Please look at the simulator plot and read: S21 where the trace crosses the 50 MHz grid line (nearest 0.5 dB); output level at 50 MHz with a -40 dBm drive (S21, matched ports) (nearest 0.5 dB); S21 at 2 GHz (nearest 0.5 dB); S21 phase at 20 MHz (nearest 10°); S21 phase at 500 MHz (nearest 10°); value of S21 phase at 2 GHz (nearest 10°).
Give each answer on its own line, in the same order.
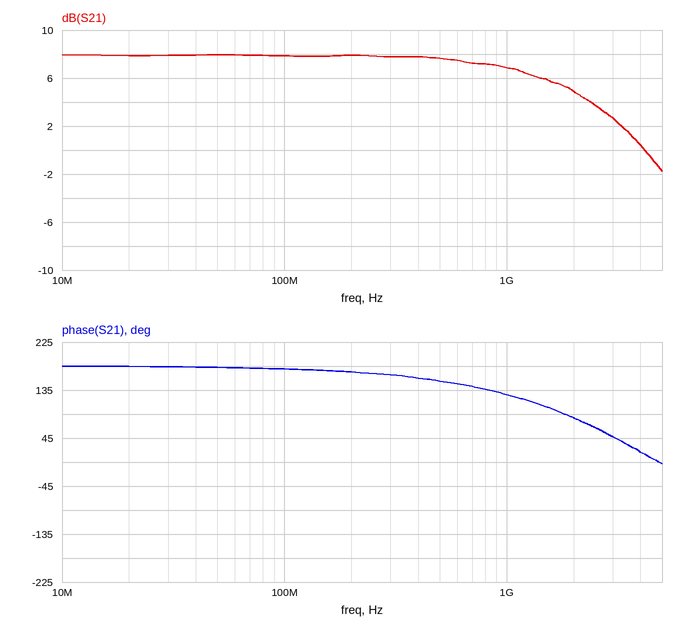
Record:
8.0 dB
-32.0 dBm
5.0 dB
180°
150°
80°
